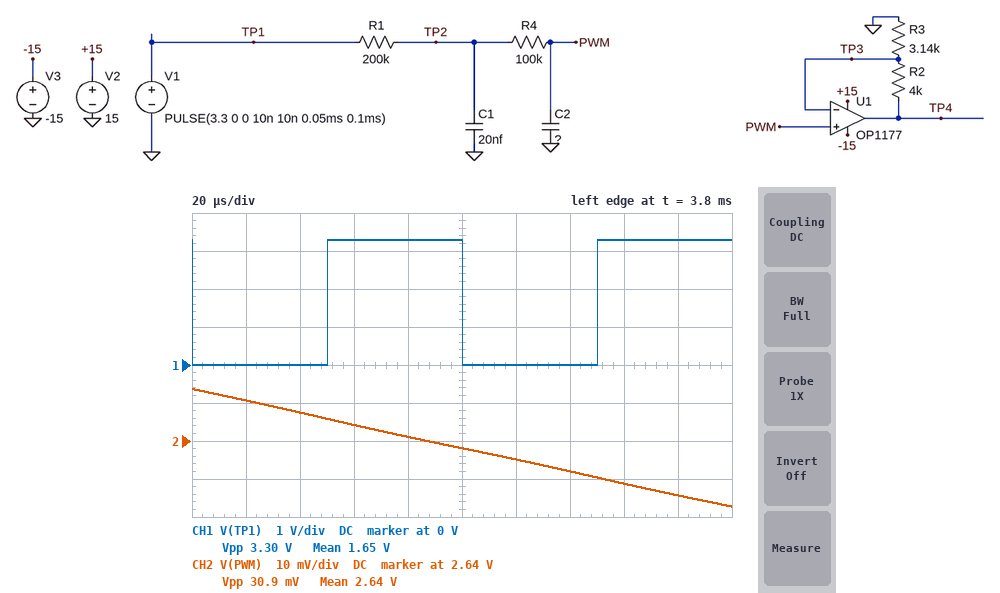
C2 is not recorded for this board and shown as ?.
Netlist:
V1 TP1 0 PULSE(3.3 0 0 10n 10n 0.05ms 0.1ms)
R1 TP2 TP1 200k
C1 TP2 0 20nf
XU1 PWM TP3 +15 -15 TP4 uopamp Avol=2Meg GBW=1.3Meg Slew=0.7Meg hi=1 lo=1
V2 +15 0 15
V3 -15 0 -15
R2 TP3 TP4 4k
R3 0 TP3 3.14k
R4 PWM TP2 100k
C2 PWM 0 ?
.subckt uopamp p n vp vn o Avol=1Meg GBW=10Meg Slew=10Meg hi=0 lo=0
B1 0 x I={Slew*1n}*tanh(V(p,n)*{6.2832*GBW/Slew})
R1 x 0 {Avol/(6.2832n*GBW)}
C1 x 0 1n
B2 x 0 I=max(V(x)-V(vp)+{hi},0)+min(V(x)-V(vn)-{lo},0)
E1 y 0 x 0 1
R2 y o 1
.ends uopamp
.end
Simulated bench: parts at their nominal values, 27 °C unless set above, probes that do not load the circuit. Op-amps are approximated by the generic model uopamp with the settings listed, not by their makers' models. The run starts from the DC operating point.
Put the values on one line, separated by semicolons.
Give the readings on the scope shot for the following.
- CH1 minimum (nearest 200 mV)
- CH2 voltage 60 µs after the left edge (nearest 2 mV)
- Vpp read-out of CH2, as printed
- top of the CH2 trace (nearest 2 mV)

0 V; 2.644 V; 30.9 mV; 2.654 V
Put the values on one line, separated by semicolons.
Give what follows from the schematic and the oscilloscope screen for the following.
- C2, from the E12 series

10 nF
